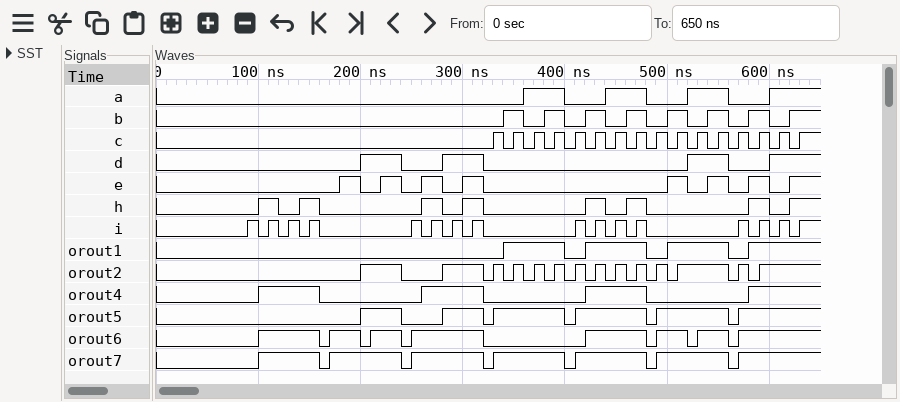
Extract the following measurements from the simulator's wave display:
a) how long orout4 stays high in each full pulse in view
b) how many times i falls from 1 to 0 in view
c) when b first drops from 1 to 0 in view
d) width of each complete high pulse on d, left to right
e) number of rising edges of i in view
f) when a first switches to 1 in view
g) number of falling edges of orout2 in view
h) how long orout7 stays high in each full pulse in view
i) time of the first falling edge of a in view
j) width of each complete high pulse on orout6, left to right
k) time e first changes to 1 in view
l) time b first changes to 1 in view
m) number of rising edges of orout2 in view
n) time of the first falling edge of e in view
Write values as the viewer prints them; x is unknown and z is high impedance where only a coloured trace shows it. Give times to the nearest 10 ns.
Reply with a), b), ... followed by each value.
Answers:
a) 60 ns, 60 ns, 60 ns
b) 15
c) 360 ns
d) 40 ns, 40 ns, 40 ns
e) 16
f) 360 ns
g) 13
h) 60 ns, 70 ns, 70 ns, 70 ns, 70 ns, 70 ns
i) 400 ns
j) 60 ns, 30 ns, 30 ns, 70 ns, 60 ns, 30 ns, 30 ns
k) 180 ns
l) 340 ns
m) 14
n) 200 ns
